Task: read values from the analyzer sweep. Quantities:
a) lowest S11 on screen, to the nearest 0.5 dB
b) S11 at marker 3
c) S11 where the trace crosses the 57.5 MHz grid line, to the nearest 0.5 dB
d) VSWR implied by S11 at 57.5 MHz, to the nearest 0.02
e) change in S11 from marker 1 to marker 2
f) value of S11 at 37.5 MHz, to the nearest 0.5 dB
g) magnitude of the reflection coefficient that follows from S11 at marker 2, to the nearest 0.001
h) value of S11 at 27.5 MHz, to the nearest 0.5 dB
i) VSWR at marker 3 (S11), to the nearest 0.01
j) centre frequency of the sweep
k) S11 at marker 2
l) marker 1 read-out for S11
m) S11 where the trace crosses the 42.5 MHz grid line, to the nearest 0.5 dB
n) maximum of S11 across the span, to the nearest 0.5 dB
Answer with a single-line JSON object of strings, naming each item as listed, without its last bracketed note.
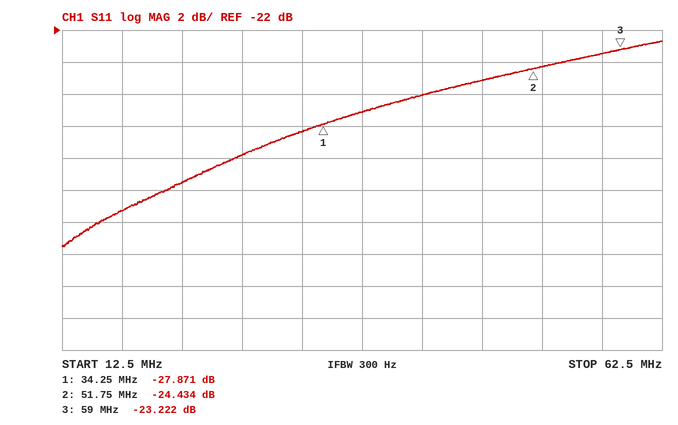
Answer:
{"lowest S11 on screen, to the nearest 0.5 dB": "-35.5 dB", "S11 at marker 3": "-23.222 dB", "S11 where the trace crosses the 57.5 MHz grid line, to the nearest 0.5 dB": "-23.5 dB", "VSWR implied by S11 at 57.5 MHz, to the nearest 0.02": "1.14", "change in S11 from marker 1 to marker 2": "3.437 dB", "value of S11 at 37.5 MHz, to the nearest 0.5 dB": "-27.0 dB", "magnitude of the reflection coefficient that follows from S11 at marker 2, to the nearest 0.001": "0.060", "value of S11 at 27.5 MHz, to the nearest 0.5 dB": "-30.0 dB", "VSWR at marker 3 (S11), to the nearest 0.01": "1.15", "centre frequency of the sweep": "37.5 MHz", "S11 at marker 2": "-24.434 dB", "marker 1 read-out for S11": "-27.871 dB", "S11 where the trace crosses the 42.5 MHz grid line, to the nearest 0.5 dB": "-26.0 dB", "maximum of S11 across the span, to the nearest 0.5 dB": "-22.5 dB"}
